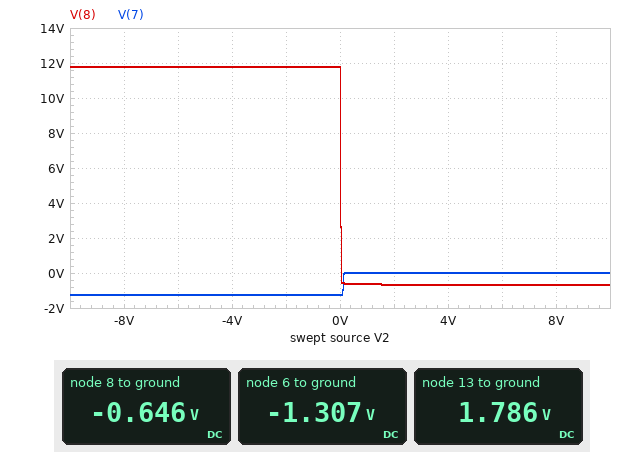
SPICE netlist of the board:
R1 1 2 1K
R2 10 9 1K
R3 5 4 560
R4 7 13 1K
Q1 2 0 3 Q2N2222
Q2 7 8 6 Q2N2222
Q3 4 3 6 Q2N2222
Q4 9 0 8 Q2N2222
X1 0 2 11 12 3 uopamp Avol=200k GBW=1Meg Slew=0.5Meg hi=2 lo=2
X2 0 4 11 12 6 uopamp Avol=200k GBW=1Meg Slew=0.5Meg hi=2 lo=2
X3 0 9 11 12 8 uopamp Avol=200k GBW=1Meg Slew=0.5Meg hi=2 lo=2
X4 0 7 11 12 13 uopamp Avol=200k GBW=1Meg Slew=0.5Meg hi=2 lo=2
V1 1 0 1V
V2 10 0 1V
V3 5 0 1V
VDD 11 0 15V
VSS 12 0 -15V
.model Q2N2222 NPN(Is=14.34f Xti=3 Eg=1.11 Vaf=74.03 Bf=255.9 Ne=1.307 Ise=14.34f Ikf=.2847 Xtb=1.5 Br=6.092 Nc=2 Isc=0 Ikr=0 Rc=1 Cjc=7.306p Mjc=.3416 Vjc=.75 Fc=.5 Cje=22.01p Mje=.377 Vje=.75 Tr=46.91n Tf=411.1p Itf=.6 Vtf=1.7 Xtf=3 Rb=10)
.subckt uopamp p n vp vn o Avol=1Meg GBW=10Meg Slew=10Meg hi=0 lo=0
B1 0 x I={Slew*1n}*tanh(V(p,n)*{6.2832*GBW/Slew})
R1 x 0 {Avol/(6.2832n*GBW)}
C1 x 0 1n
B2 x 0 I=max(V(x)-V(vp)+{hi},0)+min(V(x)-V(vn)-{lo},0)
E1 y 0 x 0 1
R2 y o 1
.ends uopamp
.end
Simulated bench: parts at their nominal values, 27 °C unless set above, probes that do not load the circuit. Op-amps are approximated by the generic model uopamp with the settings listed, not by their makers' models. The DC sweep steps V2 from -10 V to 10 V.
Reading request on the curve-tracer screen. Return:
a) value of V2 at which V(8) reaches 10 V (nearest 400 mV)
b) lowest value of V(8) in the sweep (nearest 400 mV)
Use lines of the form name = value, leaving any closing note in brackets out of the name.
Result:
value of V2 at which V(8) reaches 10 V = 0 V
lowest value of V(8) in the sweep = -800 mV
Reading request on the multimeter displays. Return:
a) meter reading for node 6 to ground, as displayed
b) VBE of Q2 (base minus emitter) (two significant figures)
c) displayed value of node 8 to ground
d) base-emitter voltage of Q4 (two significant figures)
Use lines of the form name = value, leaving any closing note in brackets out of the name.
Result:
meter reading for node 6 to ground, as displayed = -1.307 V
VBE of Q2 (base minus emitter) = 660 mV
displayed value of node 8 to ground = -0.646 V
base-emitter voltage of Q4 = 650 mV
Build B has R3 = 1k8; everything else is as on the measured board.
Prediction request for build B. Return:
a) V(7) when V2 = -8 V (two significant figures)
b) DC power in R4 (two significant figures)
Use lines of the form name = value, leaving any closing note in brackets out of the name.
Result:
V(7) when V2 = -8 V = -1.2 V
DC power in R4 = 310 µW
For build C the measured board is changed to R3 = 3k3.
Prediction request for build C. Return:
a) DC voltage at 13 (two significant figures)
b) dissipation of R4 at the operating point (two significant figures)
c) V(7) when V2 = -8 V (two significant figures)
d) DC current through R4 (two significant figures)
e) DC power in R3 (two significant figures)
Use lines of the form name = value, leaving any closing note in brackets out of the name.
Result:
DC voltage at 13 = 300 mV
dissipation of R4 at the operating point = 92 µW
V(7) when V2 = -8 V = -1.2 V
DC current through R4 = 300 µA
DC power in R3 = 300 µW
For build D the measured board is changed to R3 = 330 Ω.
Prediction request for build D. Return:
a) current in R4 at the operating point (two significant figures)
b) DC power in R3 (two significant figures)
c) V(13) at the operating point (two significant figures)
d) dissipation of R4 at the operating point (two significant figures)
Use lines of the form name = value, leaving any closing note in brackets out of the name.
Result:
current in R4 at the operating point = 3.0 mA
DC power in R3 = 3.0 mW
V(13) at the operating point = 3.0 V
dissipation of R4 at the operating point = 9.2 mW
